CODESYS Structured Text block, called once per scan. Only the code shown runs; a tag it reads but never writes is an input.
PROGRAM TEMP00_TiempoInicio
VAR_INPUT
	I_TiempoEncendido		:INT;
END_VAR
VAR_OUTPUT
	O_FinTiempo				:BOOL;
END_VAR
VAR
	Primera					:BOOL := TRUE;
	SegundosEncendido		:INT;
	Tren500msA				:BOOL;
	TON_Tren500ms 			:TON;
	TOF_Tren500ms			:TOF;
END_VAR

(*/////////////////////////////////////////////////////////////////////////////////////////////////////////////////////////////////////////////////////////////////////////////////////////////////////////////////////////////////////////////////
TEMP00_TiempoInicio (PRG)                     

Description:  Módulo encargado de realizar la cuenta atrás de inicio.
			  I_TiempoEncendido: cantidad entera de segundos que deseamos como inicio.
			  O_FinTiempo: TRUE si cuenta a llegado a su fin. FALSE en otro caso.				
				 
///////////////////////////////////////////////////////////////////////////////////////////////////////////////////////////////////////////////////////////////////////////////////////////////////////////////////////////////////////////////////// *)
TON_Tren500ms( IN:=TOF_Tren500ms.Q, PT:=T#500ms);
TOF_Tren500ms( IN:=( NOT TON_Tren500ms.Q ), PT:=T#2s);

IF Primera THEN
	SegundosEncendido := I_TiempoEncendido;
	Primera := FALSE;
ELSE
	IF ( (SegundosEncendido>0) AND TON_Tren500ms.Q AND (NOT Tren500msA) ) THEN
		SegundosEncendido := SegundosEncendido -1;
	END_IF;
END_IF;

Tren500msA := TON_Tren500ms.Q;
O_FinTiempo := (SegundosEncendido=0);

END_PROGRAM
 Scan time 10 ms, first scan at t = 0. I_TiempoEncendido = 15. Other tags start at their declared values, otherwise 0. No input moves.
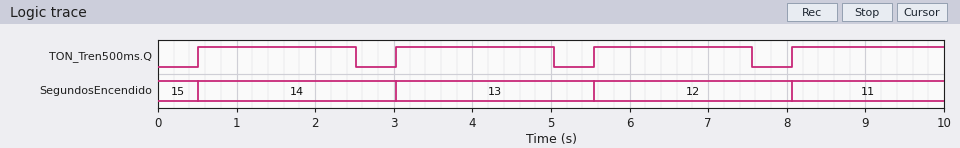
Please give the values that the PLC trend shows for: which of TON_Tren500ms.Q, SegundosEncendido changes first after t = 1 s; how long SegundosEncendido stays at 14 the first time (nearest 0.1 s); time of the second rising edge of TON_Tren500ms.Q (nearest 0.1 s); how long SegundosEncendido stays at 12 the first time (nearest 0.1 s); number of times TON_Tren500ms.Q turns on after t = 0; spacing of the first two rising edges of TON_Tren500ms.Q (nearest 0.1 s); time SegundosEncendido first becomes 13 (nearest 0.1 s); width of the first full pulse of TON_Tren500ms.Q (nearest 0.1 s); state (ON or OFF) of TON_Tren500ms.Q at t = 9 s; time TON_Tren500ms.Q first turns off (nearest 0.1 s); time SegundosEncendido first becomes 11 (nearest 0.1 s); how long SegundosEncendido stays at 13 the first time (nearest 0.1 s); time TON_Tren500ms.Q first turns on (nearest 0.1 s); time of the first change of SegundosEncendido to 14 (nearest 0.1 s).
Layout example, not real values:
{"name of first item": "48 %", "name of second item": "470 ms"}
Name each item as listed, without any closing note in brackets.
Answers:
{"which of TON_Tren500ms.Q, SegundosEncendido changes first after t = 1 s": "TON_Tren500ms.Q", "how long SegundosEncendido stays at 14 the first time": "2.5 s", "time of the second rising edge of TON_Tren500ms.Q": "3.0 s", "how long SegundosEncendido stays at 12 the first time": "2.5 s", "number of times TON_Tren500ms.Q turns on after t = 0": "4", "spacing of the first two rising edges of TON_Tren500ms.Q": "2.5 s", "time SegundosEncendido first becomes 13": "3.0 s", "width of the first full pulse of TON_Tren500ms.Q": "2.0 s", "state (ON or OFF) of TON_Tren500ms.Q at t = 9 s": "ON", "time TON_Tren500ms.Q first turns off": "2.5 s", "time SegundosEncendido first becomes 11": "8.1 s", "how long SegundosEncendido stays at 13 the first time": "2.5 s", "time TON_Tren500ms.Q first turns on": "0.5 s", "time of the first change of SegundosEncendido to 14": "0.5 s"}
